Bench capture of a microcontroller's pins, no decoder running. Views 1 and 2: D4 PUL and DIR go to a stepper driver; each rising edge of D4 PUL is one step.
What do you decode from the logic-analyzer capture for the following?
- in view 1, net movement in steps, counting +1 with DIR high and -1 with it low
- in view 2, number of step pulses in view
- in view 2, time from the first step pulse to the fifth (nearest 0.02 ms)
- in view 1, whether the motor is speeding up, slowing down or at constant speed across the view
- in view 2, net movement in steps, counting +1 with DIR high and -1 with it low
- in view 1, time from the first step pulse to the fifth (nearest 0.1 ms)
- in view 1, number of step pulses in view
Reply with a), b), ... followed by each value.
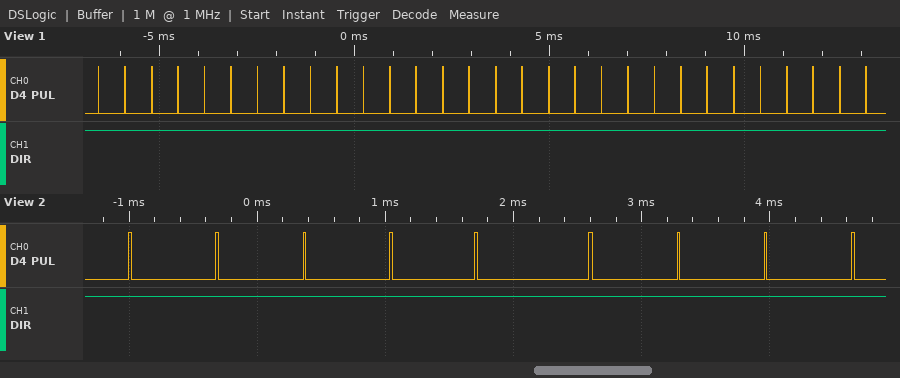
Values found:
a) +30
b) 9
c) 2.70 ms
d) constant speed
e) +9
f) 2.7 ms
g) 30
